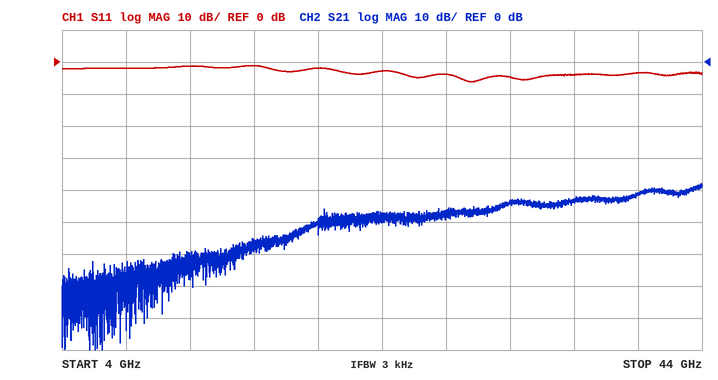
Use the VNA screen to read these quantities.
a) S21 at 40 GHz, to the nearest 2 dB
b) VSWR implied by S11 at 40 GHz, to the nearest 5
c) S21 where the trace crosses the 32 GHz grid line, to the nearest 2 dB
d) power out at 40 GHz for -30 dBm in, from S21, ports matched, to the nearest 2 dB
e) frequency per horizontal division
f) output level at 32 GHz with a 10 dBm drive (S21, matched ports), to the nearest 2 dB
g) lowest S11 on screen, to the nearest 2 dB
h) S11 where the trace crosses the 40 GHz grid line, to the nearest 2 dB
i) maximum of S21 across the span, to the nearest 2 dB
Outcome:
-42 dB
5
-44 dB
-72 dBm
4 GHz
-34 dBm
-6 dB
-4 dB
-38 dB
